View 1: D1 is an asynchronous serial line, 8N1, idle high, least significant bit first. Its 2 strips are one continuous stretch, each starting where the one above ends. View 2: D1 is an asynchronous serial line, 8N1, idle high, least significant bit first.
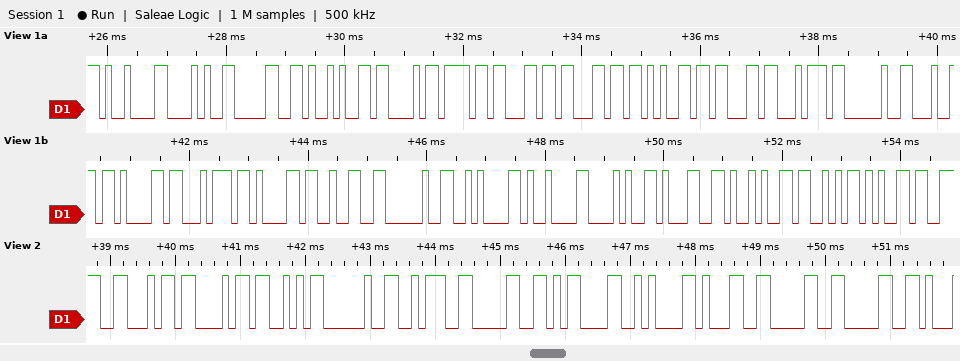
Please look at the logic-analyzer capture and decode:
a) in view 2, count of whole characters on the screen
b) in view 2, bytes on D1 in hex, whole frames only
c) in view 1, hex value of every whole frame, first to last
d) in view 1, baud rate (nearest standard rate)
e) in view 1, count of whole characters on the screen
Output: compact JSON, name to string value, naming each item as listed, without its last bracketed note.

{"in view 2, count of whole characters on the screen": "11", "in view 2, bytes on D1 in hex, whole frames only": "0x46 0x43 0x53 0x20 0x3A 0x30 0x0D 0x0A 0x31 0x30 0x30", "in view 1, hex value of every whole frame, first to last": "0x09 0x28 0x30 0x29 0x43 0x6F 0x6C 0x6C 0x65 0x63 0x74 0x20 0x64 0x61 0x74 0x61 0x32 0x20 0x0A 0x09 0x28 0x31 0x29 0x53 0x65", "in view 1, baud rate": "9600 baud", "in view 1, count of whole characters on the screen": "25"}
